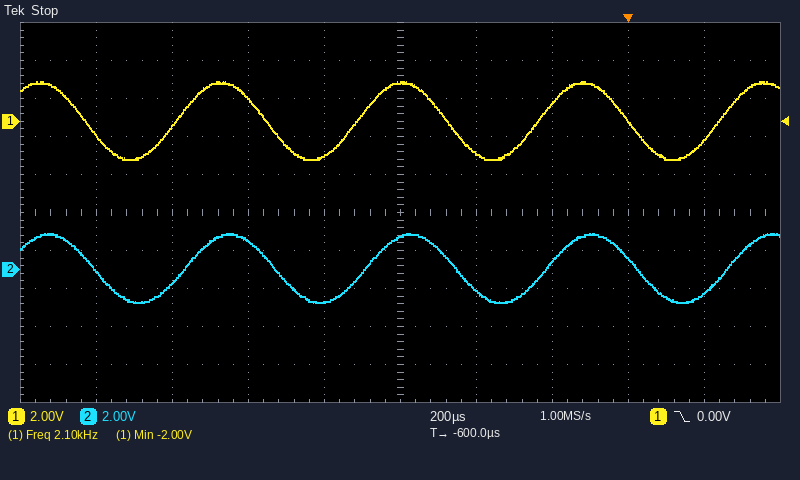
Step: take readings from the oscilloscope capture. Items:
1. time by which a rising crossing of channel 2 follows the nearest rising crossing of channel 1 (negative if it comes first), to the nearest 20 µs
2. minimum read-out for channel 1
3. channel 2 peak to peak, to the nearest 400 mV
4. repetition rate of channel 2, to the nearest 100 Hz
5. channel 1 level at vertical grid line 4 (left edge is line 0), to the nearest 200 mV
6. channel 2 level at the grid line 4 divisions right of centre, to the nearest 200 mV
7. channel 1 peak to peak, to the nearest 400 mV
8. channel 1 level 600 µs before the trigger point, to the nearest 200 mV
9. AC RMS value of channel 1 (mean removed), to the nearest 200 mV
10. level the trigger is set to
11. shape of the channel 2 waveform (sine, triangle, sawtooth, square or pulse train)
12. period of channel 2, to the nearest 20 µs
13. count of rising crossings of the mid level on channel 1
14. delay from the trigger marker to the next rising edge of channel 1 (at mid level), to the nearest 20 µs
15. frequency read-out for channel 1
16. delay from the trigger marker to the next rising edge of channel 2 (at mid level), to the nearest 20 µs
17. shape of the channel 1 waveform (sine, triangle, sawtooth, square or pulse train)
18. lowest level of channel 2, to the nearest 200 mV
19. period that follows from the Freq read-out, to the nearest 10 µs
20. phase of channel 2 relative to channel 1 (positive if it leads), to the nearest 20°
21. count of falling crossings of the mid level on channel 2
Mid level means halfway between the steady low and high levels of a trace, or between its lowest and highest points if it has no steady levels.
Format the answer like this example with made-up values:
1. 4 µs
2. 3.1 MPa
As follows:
1. +20 µs
2. -2.00 V
3. 3.6 V
4. 2.1 kHz
5. -1.8 V
6. -1.2 V
7. 4.0 V
8. 2.0 V
9. 1.4 V
10. 0.00 V
11. sine
12. 480 µs
13. 4
14. 240 µs
15. 2.10 kHz
16. 260 µs
17. sine
18. -1.8 V
19. 480 µs
20. -20°
21. 4
